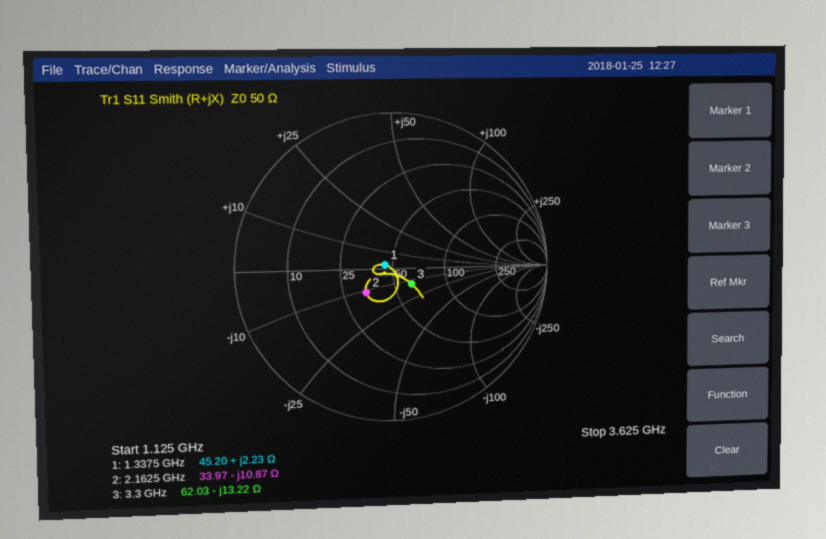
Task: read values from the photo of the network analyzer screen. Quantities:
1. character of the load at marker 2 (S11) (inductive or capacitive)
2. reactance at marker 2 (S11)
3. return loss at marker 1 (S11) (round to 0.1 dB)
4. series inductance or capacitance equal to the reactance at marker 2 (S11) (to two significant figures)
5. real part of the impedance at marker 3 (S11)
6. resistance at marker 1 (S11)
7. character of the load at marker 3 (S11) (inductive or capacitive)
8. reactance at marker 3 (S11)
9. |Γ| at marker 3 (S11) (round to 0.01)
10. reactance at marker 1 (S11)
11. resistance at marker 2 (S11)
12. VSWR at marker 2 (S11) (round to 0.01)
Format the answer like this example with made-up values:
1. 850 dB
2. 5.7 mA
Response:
1. capacitive
2. -10.87 Ω
3. 25.1 dB
4. 6.8 pF
5. 62.03 Ω
6. 45.20 Ω
7. capacitive
8. -13.22 Ω
9. 0.16
10. +2.23 Ω
11. 33.97 Ω
12. 1.59
